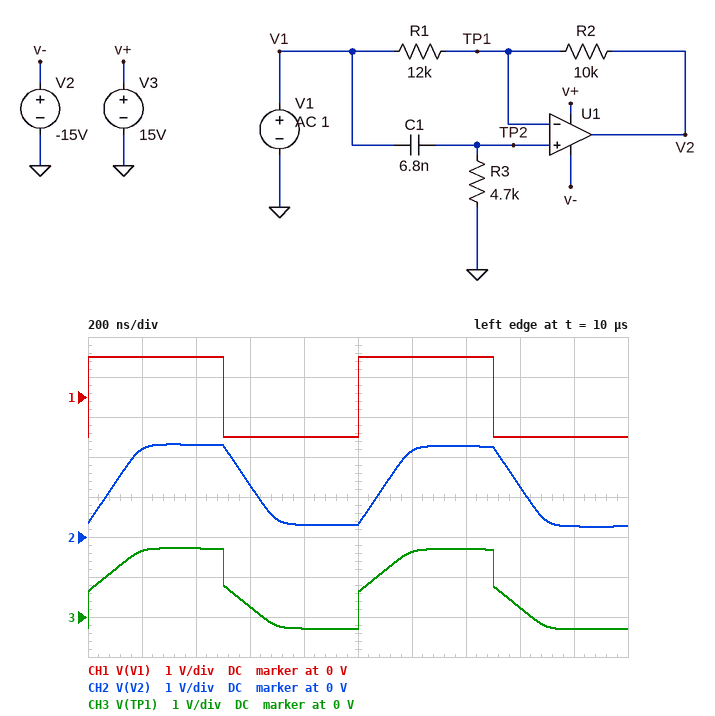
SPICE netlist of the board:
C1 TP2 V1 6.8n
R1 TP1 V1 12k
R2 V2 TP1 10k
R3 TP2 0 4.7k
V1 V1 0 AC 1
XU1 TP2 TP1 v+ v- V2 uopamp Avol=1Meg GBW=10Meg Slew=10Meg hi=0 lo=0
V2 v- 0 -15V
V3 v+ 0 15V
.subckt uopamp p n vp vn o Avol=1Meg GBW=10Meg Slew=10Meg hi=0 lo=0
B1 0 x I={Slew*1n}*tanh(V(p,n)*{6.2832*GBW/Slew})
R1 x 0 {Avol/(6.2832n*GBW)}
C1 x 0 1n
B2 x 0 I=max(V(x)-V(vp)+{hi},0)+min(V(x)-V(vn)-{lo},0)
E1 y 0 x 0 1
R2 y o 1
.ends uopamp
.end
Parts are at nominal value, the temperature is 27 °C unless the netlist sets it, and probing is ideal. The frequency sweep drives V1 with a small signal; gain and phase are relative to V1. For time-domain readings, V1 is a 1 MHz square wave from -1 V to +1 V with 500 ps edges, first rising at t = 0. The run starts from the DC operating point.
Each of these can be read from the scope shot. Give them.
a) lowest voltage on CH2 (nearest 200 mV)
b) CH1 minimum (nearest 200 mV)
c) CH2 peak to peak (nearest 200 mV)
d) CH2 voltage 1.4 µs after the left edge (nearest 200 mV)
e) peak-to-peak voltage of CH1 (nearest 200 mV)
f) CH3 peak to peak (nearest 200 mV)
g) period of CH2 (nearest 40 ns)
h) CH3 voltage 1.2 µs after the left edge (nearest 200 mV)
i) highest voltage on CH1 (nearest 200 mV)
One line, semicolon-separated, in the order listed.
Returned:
200 mV; -1.0 V; 2.0 V; 2.2 V; 2.0 V; 2.0 V; 1.00 µs; 1.6 V; 1.0 V
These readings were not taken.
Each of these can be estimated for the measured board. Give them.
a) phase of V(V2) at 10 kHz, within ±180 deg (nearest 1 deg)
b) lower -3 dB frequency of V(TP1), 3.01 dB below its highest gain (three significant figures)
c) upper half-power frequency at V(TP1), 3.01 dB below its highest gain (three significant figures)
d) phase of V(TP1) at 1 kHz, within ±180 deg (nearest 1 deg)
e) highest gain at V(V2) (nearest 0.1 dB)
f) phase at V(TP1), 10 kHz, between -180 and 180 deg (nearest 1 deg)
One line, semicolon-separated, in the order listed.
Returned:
49 deg; 4.97 kHz; 7.13 MHz; 79 deg; 0 dB; 26 deg
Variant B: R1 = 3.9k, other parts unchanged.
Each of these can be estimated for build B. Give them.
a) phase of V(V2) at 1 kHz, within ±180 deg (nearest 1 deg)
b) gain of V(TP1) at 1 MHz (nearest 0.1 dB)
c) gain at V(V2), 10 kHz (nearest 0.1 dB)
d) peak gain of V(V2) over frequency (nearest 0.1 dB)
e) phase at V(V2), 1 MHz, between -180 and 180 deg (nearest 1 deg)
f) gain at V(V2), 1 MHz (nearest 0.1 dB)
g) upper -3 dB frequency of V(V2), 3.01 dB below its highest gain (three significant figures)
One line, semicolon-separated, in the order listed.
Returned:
164 deg; -0.2 dB; 3.2 dB; 8.2 dB; -19 deg; -0.5 dB; 5.97 kHz
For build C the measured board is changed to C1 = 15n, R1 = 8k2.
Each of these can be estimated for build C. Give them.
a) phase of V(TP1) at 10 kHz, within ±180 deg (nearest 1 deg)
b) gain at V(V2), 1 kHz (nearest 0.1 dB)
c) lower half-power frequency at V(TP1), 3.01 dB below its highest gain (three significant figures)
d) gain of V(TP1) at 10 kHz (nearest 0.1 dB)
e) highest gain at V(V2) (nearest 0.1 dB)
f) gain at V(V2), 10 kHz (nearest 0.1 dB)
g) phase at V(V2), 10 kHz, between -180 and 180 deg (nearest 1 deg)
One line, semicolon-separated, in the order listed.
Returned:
13 deg; 1.5 dB; 2.26 kHz; -0.2 dB; 1.7 dB; 0.1 dB; 28 deg
